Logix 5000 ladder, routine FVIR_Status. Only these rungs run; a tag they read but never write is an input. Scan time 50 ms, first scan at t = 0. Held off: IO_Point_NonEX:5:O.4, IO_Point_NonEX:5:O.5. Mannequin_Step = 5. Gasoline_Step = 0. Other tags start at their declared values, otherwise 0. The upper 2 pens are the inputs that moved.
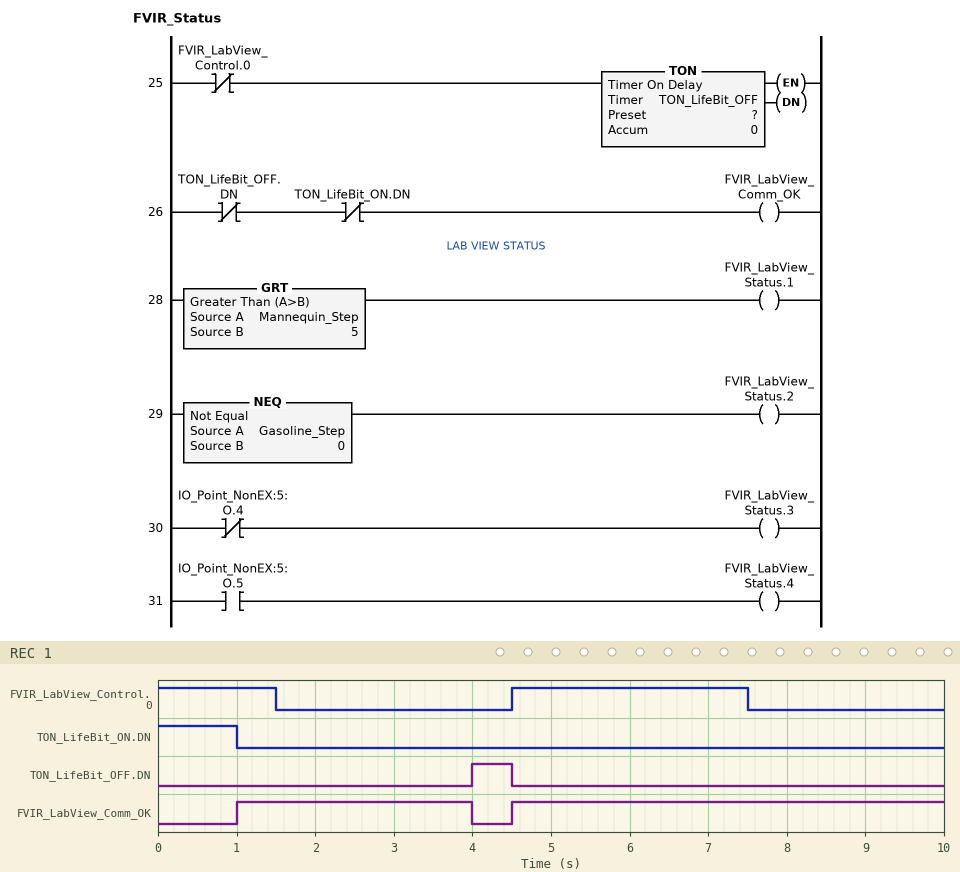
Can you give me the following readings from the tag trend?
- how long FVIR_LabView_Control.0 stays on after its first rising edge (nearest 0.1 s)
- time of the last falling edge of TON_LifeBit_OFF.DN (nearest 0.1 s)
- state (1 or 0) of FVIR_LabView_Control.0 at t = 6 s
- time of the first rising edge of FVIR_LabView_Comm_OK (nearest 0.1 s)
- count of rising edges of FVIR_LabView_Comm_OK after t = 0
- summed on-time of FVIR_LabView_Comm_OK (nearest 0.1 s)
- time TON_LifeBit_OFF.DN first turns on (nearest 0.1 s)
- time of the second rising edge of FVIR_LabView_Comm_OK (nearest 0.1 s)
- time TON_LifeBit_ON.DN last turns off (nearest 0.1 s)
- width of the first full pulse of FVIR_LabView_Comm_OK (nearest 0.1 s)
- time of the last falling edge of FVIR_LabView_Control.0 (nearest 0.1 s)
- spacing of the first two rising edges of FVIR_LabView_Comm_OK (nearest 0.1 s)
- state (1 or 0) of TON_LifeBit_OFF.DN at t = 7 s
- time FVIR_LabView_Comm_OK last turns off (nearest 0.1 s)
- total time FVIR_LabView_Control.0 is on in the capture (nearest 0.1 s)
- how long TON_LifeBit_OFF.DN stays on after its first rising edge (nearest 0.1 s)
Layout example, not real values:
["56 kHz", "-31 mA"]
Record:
["3.0 s", "4.5 s", "1", "1.0 s", "2", "8.5 s", "4.0 s", "4.5 s", "1.0 s", "3.0 s", "7.5 s", "3.5 s", "0", "4.0 s", "4.5 s", "0.5 s"]
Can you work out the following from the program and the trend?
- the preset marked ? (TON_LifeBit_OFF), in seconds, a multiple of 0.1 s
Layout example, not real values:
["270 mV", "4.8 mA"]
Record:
["2.5 s"]
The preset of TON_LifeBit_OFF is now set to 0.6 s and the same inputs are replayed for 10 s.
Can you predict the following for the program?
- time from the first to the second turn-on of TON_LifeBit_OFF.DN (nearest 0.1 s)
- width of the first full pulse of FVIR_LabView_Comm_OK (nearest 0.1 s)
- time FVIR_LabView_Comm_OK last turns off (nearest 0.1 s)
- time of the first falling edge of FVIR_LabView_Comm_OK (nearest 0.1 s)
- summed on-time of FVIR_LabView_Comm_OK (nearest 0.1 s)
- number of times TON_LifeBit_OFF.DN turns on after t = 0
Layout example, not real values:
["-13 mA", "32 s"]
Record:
["6.0 s", "1.1 s", "8.1 s", "2.1 s", "4.7 s", "2"]
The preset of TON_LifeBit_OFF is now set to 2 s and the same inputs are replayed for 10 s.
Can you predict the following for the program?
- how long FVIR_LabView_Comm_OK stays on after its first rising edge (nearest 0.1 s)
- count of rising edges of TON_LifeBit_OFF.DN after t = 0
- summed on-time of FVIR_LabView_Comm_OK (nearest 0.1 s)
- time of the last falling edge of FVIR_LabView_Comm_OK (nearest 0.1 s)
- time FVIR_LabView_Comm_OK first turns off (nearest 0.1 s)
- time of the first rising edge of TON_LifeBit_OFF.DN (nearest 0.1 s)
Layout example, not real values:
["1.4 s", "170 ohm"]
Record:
["2.5 s", "2", "7.5 s", "9.5 s", "3.5 s", "3.5 s"]
